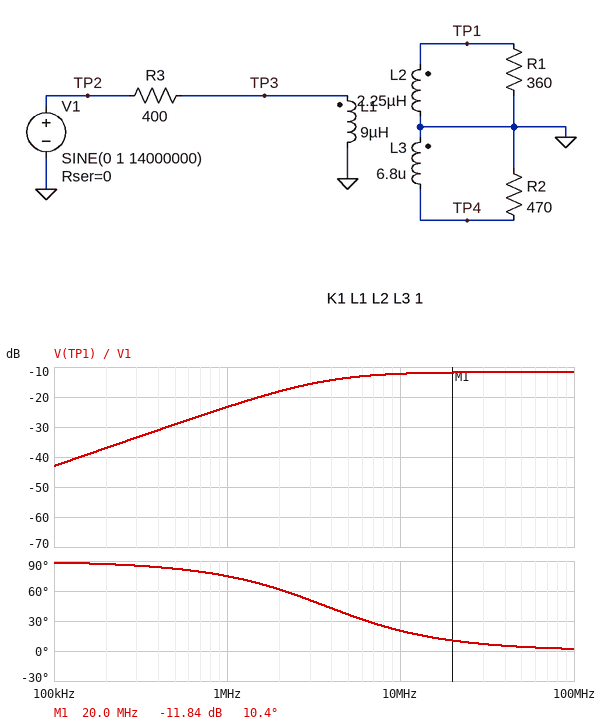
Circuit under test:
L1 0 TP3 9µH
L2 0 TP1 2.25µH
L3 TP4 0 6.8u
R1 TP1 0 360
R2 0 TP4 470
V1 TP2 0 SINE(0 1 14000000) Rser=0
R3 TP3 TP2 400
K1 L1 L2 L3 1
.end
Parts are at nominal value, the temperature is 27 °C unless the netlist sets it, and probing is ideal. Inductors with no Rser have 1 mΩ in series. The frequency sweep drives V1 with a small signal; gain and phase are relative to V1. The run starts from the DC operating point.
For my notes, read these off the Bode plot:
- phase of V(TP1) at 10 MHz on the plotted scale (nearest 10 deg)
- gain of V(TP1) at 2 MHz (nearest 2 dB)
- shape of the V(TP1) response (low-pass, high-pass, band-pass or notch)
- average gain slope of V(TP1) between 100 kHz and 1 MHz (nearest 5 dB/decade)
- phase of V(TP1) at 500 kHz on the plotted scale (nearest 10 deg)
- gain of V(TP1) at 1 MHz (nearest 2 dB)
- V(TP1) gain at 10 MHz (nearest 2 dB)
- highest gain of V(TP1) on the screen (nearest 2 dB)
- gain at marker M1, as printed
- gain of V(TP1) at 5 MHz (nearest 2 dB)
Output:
20 deg
-18 dB
high-pass
20 dB/decade
80 deg
-24 dB
-12 dB
-12 dB
-11.84 dB
-14 dB
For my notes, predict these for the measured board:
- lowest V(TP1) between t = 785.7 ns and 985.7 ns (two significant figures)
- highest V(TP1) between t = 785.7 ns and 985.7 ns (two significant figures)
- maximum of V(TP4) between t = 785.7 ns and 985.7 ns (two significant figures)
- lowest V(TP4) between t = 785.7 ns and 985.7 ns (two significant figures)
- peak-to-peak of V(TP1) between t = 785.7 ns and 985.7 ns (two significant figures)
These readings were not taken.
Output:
-250 mV
250 mV
440 mV
-440 mV
500 mV
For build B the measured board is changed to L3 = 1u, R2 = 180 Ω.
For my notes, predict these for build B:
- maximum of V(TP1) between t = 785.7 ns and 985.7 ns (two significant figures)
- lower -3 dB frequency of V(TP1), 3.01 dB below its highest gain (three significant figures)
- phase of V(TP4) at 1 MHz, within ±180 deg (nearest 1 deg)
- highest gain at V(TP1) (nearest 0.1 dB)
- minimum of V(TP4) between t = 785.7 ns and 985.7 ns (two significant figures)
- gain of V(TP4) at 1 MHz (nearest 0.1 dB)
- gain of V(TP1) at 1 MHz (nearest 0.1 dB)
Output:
310 mV
4.64 MHz
-102 deg
-9.7 dB
-210 mV
-26.7 dB
-23.2 dB
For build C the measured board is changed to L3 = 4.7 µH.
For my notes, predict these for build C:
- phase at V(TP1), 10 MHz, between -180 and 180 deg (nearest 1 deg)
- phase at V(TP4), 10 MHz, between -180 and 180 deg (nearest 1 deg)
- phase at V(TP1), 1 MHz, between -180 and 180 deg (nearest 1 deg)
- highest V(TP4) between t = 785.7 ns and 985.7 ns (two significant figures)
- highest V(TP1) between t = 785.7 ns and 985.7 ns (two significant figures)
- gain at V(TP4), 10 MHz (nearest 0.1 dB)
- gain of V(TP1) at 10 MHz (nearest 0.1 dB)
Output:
22 deg
-158 deg
76 deg
400 mV
280 mV
-8.2 dB
-11.4 dB
